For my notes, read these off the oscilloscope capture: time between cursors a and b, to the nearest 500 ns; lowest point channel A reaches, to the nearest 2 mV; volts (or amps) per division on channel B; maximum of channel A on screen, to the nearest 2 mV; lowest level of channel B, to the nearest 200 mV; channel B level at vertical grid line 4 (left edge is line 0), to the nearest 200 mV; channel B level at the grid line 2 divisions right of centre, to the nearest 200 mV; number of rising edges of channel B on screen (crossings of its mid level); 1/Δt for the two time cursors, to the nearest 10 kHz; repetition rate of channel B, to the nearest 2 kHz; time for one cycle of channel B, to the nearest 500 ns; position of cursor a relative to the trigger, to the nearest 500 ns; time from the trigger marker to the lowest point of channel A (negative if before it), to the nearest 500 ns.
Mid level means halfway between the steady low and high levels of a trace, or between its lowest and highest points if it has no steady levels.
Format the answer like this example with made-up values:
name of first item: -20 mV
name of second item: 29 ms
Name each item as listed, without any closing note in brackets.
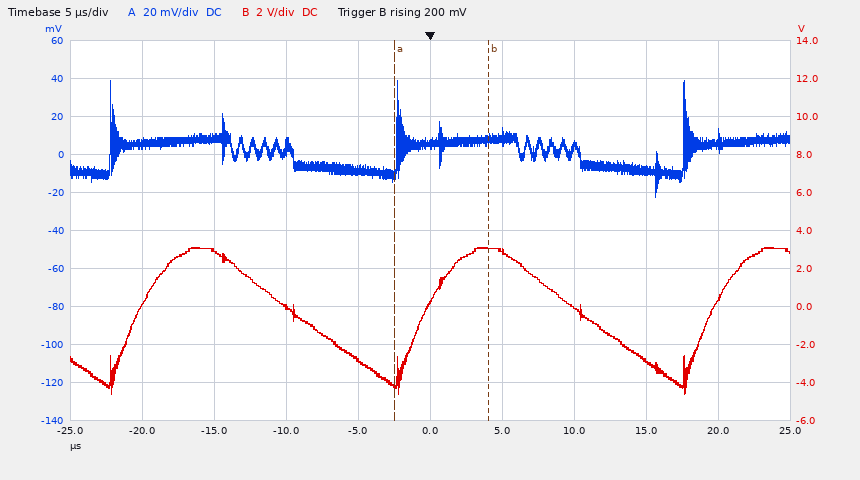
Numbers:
time between cursors a and b, to the nearest 500 ns: 6.5 µs
lowest point channel A reaches, to the nearest 2 mV: -22 mV
volts (or amps) per division on channel B: 2 V
maximum of channel A on screen, to the nearest 2 mV: 38 mV
lowest level of channel B, to the nearest 200 mV: -4.6 V
channel B level at vertical grid line 4 (left edge is line 0), to the nearest 200 mV: -2.8 V
channel B level at the grid line 2 divisions right of centre, to the nearest 200 mV: 0.0 V
number of rising edges of channel B on screen: 3
1/Δt for the two time cursors, to the nearest 10 kHz: 150 kHz
repetition rate of channel B, to the nearest 2 kHz: 50 kHz
time for one cycle of channel B, to the nearest 500 ns: 20.0 µs
position of cursor a relative to the trigger, to the nearest 500 ns: -2.5 µs
time from the trigger marker to the lowest point of channel A (negative if before it), to the nearest 500 ns: +15.5 µs
